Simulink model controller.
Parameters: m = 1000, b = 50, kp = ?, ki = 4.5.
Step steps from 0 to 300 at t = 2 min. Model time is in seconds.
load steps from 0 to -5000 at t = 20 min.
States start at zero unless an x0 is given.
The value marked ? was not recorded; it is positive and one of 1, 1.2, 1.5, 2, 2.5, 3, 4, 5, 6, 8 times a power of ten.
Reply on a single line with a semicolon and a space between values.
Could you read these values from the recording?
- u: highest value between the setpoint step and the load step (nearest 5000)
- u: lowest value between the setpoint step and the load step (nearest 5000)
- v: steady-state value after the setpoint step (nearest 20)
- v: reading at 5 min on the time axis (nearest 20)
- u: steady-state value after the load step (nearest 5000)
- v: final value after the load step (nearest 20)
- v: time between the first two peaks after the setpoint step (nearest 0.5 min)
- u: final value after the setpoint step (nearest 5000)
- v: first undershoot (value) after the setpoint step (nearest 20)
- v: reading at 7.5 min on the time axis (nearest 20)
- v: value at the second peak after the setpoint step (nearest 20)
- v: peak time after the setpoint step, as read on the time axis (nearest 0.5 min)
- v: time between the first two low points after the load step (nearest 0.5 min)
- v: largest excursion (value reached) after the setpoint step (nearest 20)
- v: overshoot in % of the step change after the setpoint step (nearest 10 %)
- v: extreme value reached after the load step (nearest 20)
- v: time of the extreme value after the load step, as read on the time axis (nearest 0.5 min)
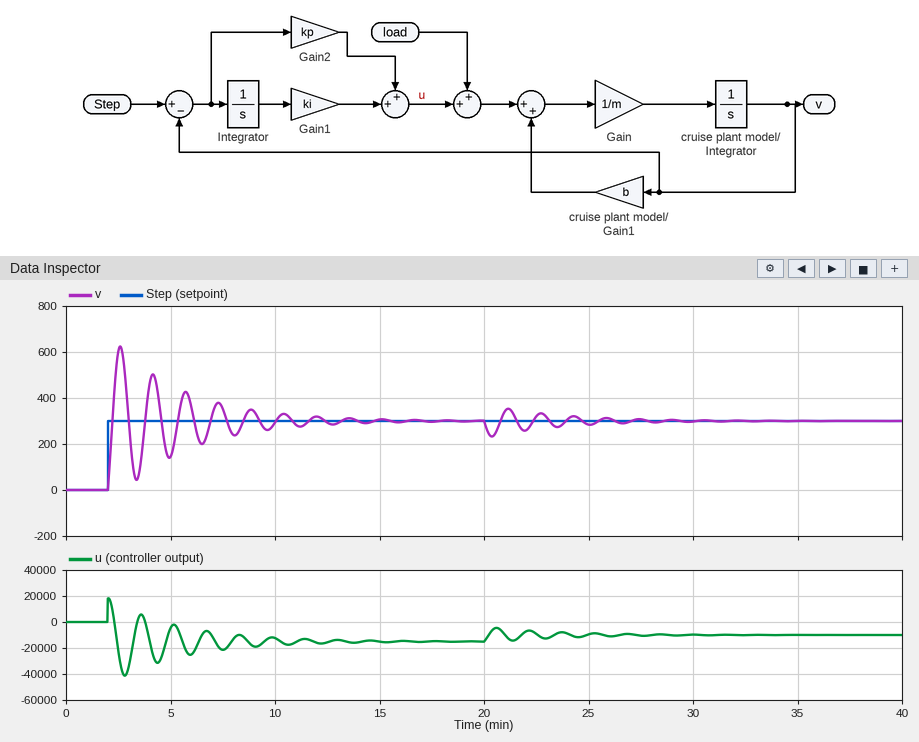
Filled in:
20000; -40000; 300; 140; -10000; 300; 1.5 min; -15000; 40; 360; 500; 2.5 min; 1.5 min; 620; 110 %; 240; 20.5 min
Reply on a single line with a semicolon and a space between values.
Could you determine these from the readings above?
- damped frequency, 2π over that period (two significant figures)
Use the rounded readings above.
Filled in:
4.2 rad/min
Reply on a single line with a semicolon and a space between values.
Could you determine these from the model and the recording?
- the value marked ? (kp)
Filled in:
60
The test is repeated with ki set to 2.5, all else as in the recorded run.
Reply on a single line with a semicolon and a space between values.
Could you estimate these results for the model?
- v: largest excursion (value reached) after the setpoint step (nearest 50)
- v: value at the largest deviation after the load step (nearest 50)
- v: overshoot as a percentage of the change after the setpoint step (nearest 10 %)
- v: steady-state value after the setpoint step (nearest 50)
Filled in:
650; 200; 120 %; 300
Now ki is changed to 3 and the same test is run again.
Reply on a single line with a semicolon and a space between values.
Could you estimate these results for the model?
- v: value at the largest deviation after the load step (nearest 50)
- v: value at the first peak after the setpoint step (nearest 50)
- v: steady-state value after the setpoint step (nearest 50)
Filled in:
200; 650; 300
